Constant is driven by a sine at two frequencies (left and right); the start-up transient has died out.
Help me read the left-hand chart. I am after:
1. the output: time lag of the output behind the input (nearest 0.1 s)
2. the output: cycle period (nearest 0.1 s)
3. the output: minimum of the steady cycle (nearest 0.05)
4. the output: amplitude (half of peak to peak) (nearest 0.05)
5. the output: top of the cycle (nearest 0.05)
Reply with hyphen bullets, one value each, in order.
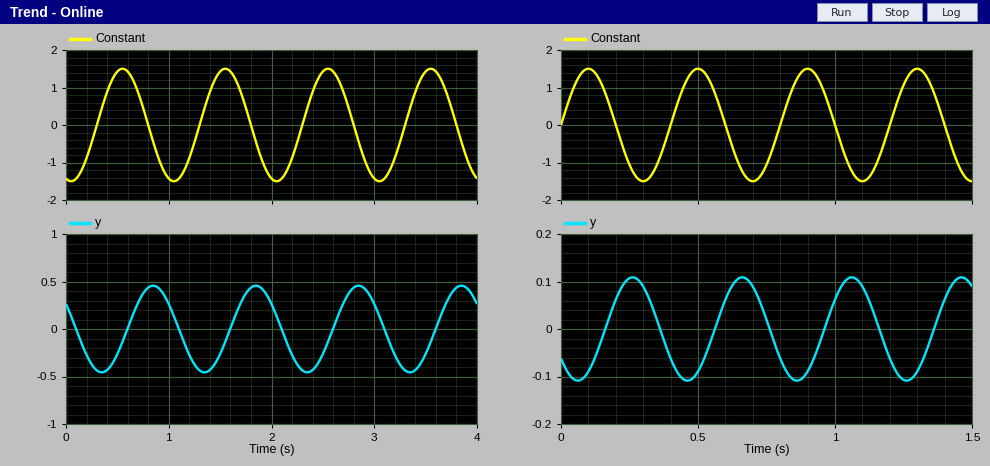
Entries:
- 0.3 s
- 1.0 s
- -0.45
- 0.45
- 0.45
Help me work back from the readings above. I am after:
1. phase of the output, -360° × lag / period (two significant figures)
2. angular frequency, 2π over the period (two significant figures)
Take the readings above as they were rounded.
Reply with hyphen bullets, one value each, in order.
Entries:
- -110°
- 6.3 rad/s
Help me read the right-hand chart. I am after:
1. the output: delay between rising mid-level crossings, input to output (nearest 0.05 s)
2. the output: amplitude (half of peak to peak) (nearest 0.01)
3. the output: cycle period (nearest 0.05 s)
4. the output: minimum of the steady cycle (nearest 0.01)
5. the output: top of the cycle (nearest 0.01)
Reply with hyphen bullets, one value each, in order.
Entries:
- 0.15 s
- 0.11
- 0.40 s
- -0.11
- 0.11
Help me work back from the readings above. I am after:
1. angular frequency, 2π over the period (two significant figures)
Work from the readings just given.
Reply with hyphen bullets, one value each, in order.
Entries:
- 16 rad/s
